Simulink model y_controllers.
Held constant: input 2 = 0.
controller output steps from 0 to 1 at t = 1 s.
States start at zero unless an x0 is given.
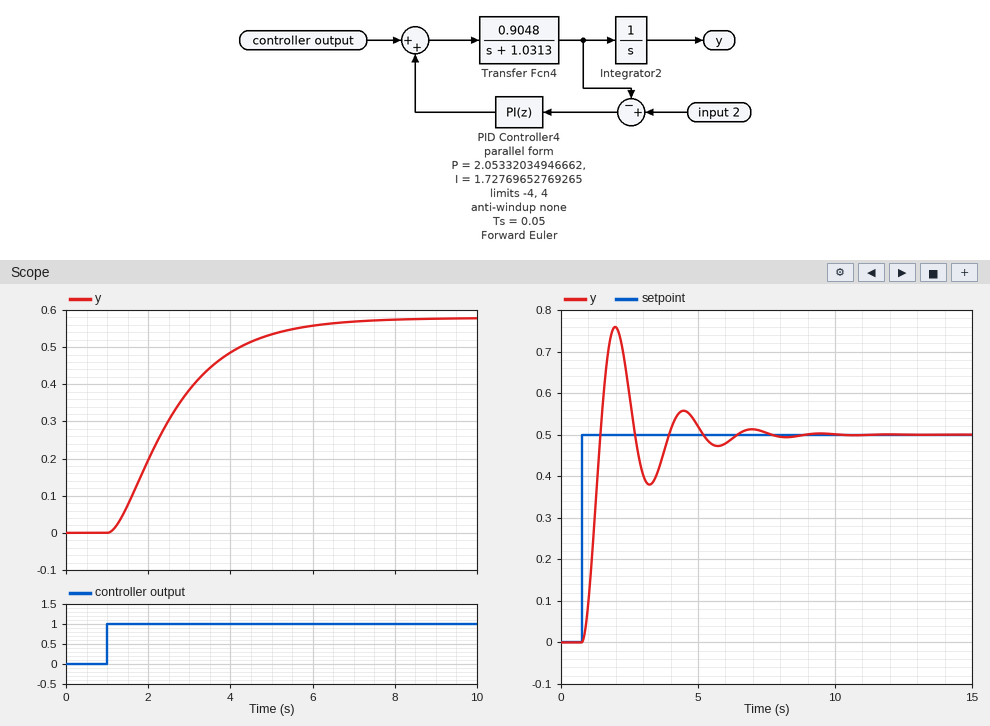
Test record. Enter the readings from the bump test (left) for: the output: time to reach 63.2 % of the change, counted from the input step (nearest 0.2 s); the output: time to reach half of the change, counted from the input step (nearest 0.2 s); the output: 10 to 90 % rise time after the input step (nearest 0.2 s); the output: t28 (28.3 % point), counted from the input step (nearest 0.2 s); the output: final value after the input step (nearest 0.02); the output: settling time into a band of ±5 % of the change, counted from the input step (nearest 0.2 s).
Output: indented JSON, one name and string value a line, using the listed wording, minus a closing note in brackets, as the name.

{
  "the output: time to reach 63.2 % of the change, counted from the input step": "1.8 s",
  "the output: time to reach half of the change, counted from the input step": "1.4 s",
  "the output: 10 to 90 % rise time after the input step": "3.2 s",
  "the output: t28 (28.3 % point), counted from the input step": "0.8 s",
  "the output: final value after the input step": "0.58",
  "the output: settling time into a band of ±5 % of the change, counted from the input step": "4.6 s"
}
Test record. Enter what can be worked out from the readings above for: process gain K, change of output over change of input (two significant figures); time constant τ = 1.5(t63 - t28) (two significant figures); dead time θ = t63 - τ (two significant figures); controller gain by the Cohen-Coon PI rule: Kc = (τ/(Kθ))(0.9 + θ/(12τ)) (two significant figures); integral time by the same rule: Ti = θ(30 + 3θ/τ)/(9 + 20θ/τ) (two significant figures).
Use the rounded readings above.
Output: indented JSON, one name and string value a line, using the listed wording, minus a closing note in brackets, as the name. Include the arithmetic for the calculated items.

{
  "process gain K, change of output over change of input": "(0.58 - 0) / 1 = 0.58",
  "time constant τ = 1.5(t63 - t28)": "1.5 × (1.8 - 0.8) = 1.5 s",
  "dead time θ = t63 - τ": "1.8 - 1.5 = 0.30 s",
  "controller gain by the Cohen-Coon PI rule: Kc = (τ/(Kθ))(0.9 + θ/(12τ))": "1.5 / (0.58 × 0.3) × (0.9 + 0.3 / (12 × 1.5)) = 7.9",
  "integral time by the same rule: Ti = θ(30 + 3θ/τ)/(9 + 20θ/τ)": "0.3 × (30 + 3 × 0.3 / 1.5) / (9 + 20 × 0.3 / 1.5) = 0.71 s"
}
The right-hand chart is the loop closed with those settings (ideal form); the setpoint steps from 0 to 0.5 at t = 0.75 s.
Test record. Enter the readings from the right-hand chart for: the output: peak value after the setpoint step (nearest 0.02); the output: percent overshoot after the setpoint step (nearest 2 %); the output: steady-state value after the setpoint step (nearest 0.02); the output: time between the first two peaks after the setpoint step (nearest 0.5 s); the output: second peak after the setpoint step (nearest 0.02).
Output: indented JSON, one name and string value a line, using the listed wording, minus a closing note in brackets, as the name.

{
  "the output: peak value after the setpoint step": "0.76",
  "the output: percent overshoot after the setpoint step": "52 %",
  "the output: steady-state value after the setpoint step": "0.50",
  "the output: time between the first two peaks after the setpoint step": "2.5 s",
  "the output: second peak after the setpoint step": "0.56"
}
